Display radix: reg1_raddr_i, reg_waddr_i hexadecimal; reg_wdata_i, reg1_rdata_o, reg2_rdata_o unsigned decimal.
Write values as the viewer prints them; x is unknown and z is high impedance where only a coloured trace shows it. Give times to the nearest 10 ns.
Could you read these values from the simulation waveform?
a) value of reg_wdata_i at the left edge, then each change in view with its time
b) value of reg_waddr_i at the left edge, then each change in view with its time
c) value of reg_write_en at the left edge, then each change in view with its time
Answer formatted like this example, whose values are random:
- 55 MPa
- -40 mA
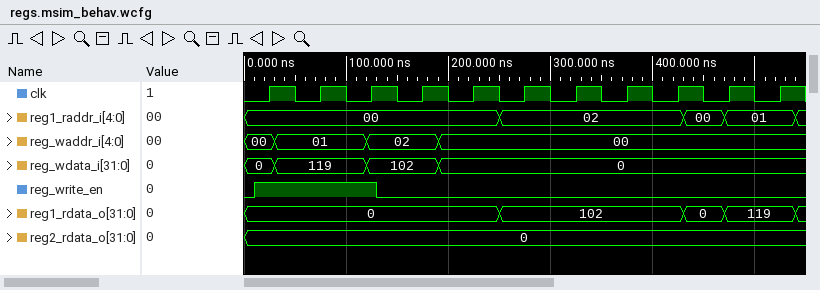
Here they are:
- 0, 119 at 30 ns, 102 at 120 ns, 0 at 190 ns
- 00, 01 at 30 ns, 02 at 120 ns, 00 at 190 ns
- 0, 1 at 10 ns, 0 at 130 ns
